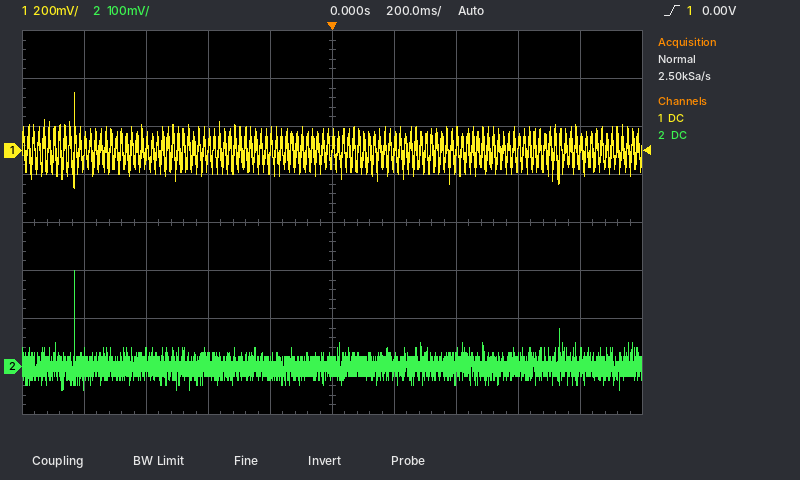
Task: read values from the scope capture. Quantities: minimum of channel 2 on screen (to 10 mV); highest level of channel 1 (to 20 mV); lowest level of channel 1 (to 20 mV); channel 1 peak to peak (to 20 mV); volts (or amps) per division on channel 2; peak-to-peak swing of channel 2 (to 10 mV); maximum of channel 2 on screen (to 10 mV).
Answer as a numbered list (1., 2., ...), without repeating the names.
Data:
1. -50 mV
2. 240 mV
3. -160 mV
4. 400 mV
5. 100 mV
6. 250 mV
7. 200 mV
